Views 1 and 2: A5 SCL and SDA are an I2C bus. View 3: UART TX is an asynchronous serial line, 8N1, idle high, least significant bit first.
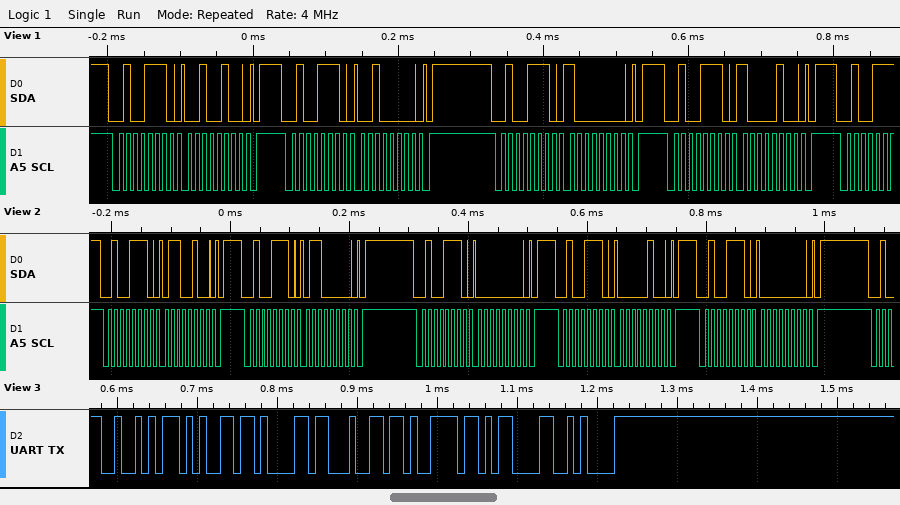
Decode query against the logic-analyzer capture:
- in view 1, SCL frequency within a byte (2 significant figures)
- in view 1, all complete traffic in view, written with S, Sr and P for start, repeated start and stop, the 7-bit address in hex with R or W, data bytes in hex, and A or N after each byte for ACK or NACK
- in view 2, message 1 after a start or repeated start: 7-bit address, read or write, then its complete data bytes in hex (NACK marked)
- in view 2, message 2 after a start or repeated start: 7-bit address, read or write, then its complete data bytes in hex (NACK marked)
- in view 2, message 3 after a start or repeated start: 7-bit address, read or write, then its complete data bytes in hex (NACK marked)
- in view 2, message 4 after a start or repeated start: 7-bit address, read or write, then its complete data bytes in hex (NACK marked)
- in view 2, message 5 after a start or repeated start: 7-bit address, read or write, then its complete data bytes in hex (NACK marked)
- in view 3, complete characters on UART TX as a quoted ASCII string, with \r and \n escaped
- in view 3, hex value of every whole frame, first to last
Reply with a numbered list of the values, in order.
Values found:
1. 100 kHz
2. S 27W A 24 A P S 27W A 20 A P S 27W A 80 A P S 27W A 84 A P
3. 0x27 write: 64
4. 0x27 write: 60
5. 0x27 write: 00
6. 0x27 write: 04
7. 0x27 write: 00
8. "Ready\r\n"
9. 52 65 61 64 79 0D 0A
